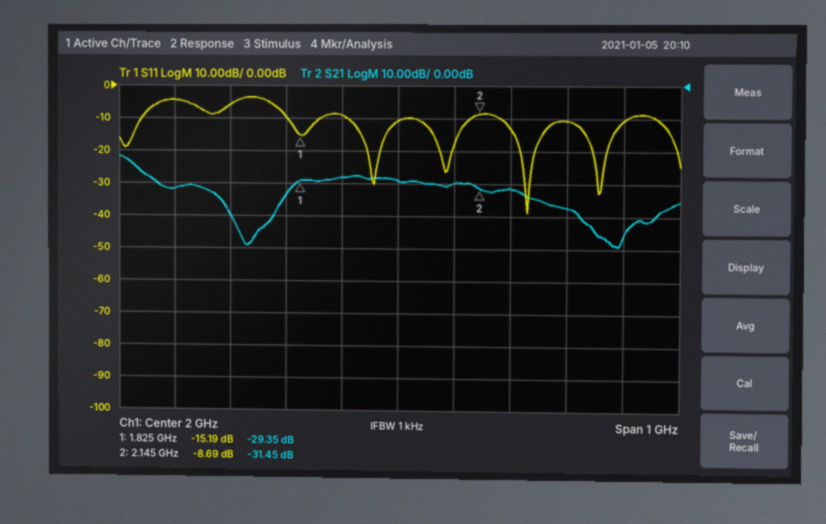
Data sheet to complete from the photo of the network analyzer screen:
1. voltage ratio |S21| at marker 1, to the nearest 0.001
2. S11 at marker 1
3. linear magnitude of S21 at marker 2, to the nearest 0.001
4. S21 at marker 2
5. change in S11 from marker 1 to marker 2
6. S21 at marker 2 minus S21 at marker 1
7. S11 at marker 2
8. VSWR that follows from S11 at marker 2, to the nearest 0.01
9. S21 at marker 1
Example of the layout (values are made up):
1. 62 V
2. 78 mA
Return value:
1. 0.034
2. -15.19 dB
3. 0.027
4. -31.45 dB
5. 6.50 dB
6. -2.10 dB
7. -8.69 dB
8. 2.16
9. -29.35 dB
